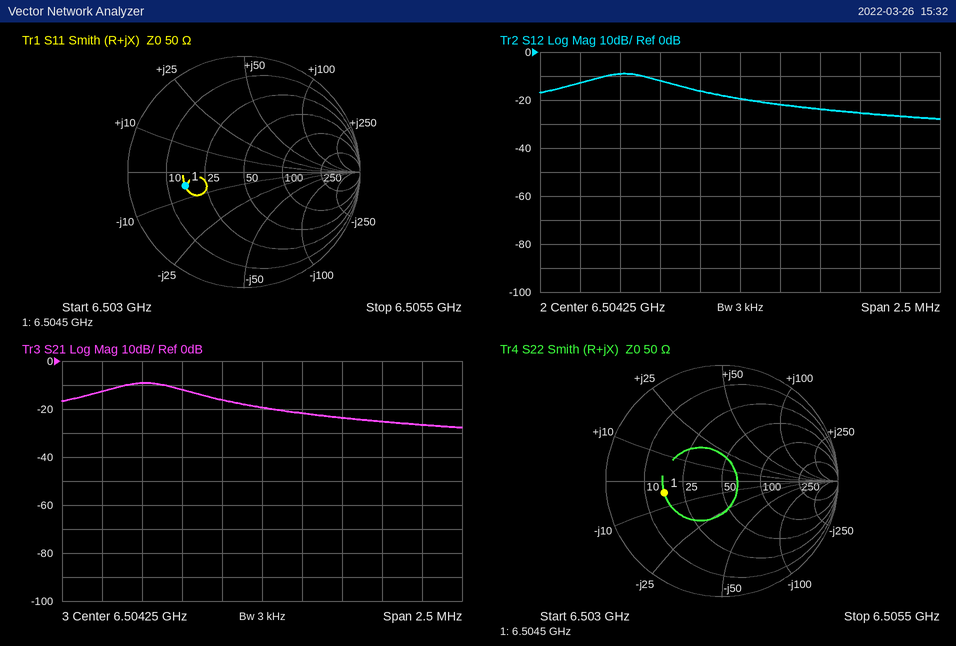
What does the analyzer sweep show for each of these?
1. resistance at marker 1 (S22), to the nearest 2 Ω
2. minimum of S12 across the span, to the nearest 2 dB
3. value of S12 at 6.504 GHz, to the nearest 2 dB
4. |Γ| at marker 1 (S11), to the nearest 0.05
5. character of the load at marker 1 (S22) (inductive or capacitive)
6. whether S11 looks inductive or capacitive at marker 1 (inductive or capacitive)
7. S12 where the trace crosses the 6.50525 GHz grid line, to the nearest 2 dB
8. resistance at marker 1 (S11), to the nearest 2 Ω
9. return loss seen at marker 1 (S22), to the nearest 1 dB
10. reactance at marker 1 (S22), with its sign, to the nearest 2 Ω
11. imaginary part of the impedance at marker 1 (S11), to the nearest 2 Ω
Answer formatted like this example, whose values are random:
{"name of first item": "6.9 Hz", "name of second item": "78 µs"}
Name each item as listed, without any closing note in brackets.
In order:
{"resistance at marker 1 (S22), to the nearest 2 Ω": "16 Ω", "minimum of S12 across the span, to the nearest 2 dB": "-28 dB", "value of S12 at 6.504 GHz, to the nearest 2 dB": "-16 dB", "|Γ| at marker 1 (S11), to the nearest 0.05": "0.50", "character of the load at marker 1 (S22)": "capacitive", "whether S11 looks inductive or capacitive at marker 1": "capacitive", "S12 where the trace crosses the 6.50525 GHz grid line, to the nearest 2 dB": "-26 dB", "resistance at marker 1 (S11), to the nearest 2 Ω": "16 Ω", "return loss seen at marker 1 (S22), to the nearest 1 dB": "6 dB", "reactance at marker 1 (S22), with its sign, to the nearest 2 Ω": "-4 Ω", "imaginary part of the impedance at marker 1 (S11), to the nearest 2 Ω": "-6 Ω"}
